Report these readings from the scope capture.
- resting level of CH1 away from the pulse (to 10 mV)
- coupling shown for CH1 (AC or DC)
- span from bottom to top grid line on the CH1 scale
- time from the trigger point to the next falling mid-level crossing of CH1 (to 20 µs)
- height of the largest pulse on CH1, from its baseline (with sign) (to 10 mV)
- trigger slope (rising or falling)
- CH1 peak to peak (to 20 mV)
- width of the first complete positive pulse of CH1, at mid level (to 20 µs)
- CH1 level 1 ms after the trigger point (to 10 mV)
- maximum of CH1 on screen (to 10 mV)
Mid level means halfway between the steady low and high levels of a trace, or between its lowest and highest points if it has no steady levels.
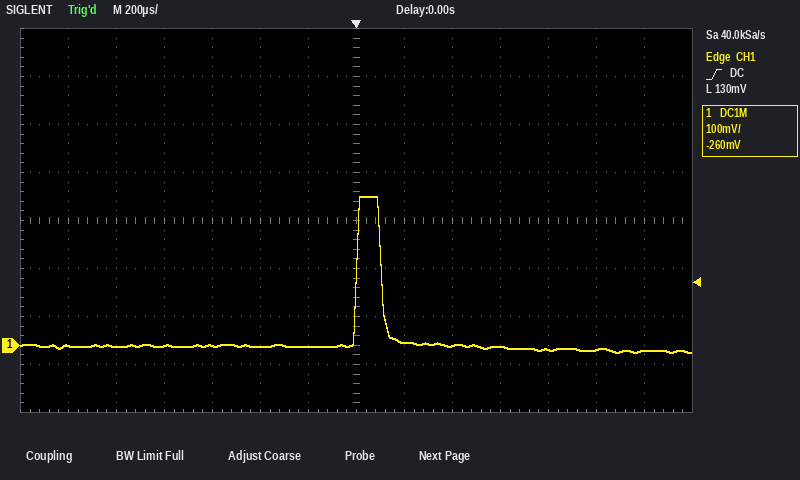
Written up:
0 mV
DC
800 mV
100 µs
+310 mV
rising
320 mV
100 µs
-10 mV
310 mV
